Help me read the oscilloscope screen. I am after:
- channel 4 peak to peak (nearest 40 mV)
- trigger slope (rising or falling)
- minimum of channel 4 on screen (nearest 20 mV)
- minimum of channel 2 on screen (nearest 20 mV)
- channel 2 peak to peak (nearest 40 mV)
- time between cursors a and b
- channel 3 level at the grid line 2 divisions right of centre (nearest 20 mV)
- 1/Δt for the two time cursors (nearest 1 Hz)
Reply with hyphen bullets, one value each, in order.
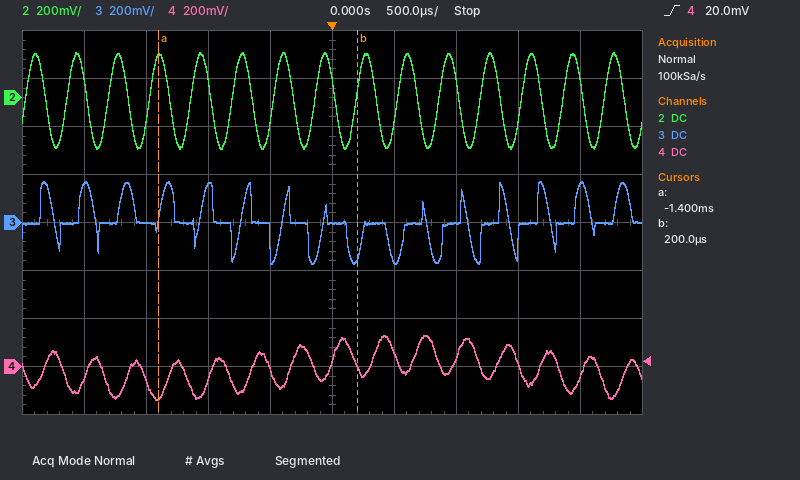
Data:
- 280 mV
- rising
- -140 mV
- -220 mV
- 400 mV
- 1.60 ms
- 0 mV
- 625 Hz
